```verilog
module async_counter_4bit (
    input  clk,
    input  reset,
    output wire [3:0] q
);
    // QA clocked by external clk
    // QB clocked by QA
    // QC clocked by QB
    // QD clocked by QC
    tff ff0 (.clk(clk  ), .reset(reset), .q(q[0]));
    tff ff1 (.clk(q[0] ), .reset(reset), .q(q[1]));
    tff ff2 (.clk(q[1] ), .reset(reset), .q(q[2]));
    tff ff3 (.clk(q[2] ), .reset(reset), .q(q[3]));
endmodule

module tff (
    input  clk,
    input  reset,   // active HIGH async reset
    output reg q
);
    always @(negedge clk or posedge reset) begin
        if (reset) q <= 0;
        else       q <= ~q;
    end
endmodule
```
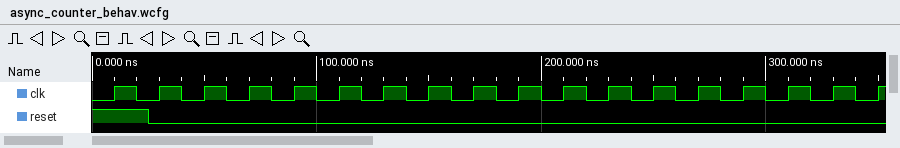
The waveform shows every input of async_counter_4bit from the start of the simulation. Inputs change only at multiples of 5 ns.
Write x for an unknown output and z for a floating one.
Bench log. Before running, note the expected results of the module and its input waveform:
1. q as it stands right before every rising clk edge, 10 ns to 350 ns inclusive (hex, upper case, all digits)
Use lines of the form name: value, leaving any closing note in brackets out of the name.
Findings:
q as it stands right before every rising clk edge, 10 ns to 350 ns inclusive: 0, 0, 1, 2, 3, 4, 5, 6, 7, 8, 9, A, B, C, D, E, F, 0
